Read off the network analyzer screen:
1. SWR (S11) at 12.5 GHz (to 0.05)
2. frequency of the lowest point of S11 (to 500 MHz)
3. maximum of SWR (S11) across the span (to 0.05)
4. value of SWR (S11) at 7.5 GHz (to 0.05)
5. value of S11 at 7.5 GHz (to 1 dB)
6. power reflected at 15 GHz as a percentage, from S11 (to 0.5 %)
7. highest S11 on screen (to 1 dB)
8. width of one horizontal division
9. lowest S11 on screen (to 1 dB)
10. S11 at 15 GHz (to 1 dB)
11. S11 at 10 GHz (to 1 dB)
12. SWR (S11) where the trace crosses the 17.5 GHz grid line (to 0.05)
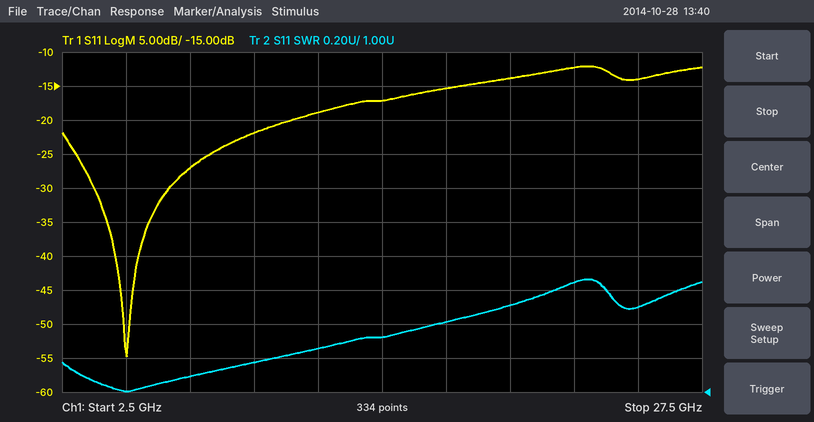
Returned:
1.25
5.0 GHz
1.65
1.10
-27 dB
2.0 %
-12 dB
2.5 GHz
-55 dB
-17 dB
-22 dB
1.40
